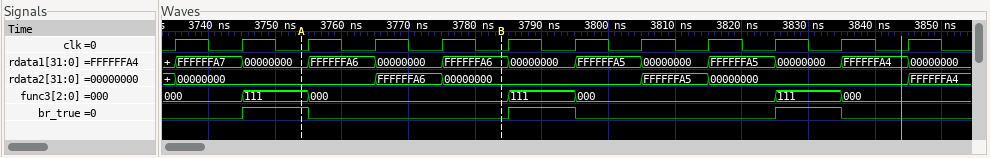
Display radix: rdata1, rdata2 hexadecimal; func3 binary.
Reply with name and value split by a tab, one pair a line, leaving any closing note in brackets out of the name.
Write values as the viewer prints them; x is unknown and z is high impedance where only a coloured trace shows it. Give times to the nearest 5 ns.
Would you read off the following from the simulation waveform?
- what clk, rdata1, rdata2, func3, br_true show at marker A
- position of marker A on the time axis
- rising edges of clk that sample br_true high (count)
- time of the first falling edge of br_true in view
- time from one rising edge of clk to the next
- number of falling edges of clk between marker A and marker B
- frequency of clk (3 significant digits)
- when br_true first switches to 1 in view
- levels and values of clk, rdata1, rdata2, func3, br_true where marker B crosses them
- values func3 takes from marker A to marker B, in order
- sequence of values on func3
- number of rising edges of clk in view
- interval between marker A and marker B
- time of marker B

what clk, rdata1, rdata2, func3, br_true show at marker A	clk=0, rdata1=00000000, rdata2=00000000, func3=111, br_true=1
position of marker A on the time axis	3755 ns
rising edges of clk that sample br_true high	3
time of the first falling edge of br_true in view	3755 ns
time from one rising edge of clk to the next	10 ns
number of falling edges of clk between marker A and marker B	3
frequency of clk	100 MHz
when br_true first switches to 1 in view	3745 ns
levels and values of clk, rdata1, rdata2, func3, br_true where marker B crosses them	clk=0, rdata1=FFFFFFA6, rdata2=00000000, func3=000, br_true=0
values func3 takes from marker A to marker B, in order	111, 000
sequence of values on func3	000, 111, 000, 111, 000, 111, 000
number of rising edges of clk in view	12
interval between marker A and marker B	30 ns
time of marker B	3785 ns
